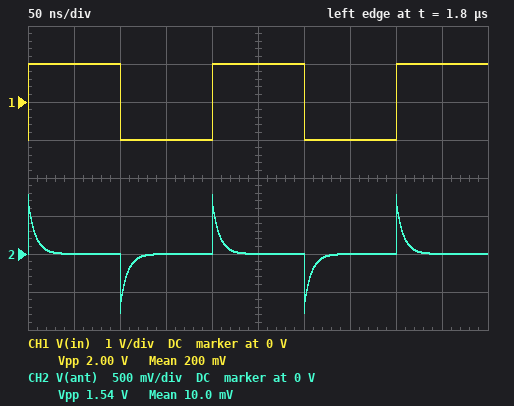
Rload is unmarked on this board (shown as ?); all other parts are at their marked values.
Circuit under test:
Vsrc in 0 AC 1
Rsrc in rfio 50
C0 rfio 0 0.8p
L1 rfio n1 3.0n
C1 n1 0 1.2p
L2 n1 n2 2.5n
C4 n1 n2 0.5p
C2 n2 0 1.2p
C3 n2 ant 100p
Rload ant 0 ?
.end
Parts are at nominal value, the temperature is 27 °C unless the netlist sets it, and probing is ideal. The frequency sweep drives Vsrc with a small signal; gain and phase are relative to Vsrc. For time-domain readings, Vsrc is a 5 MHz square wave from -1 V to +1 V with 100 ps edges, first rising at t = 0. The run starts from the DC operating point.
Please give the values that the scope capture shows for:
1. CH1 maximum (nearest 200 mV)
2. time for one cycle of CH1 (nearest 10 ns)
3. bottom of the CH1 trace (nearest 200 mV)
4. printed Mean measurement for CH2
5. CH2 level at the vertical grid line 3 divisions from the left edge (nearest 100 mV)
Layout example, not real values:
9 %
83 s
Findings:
1.0 V
200 ns
-1.0 V
10.0 mV
0 V
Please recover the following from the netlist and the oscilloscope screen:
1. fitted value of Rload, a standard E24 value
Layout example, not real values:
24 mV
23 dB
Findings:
27 Ω
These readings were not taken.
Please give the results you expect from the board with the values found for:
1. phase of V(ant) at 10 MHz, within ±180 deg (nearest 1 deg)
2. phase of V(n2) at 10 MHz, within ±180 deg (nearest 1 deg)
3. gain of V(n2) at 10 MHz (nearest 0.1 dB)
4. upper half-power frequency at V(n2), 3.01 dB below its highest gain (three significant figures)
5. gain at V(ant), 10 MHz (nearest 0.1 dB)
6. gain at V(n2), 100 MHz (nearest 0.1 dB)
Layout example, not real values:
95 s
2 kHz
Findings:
64 deg
-17 deg
-0.8 dB
23.7 MHz
-16.3 dB
-8.0 dB
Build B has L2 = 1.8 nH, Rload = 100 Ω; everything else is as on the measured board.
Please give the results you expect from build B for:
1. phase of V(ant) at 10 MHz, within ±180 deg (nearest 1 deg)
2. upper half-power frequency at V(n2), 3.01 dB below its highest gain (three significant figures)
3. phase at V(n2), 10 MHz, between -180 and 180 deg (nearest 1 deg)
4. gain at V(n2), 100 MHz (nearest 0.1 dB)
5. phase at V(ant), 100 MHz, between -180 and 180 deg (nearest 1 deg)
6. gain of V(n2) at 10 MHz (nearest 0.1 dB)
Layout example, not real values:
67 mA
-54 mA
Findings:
46 deg
31.4 MHz
-12 deg
-3.5 dB
1 deg
-1.3 dB
